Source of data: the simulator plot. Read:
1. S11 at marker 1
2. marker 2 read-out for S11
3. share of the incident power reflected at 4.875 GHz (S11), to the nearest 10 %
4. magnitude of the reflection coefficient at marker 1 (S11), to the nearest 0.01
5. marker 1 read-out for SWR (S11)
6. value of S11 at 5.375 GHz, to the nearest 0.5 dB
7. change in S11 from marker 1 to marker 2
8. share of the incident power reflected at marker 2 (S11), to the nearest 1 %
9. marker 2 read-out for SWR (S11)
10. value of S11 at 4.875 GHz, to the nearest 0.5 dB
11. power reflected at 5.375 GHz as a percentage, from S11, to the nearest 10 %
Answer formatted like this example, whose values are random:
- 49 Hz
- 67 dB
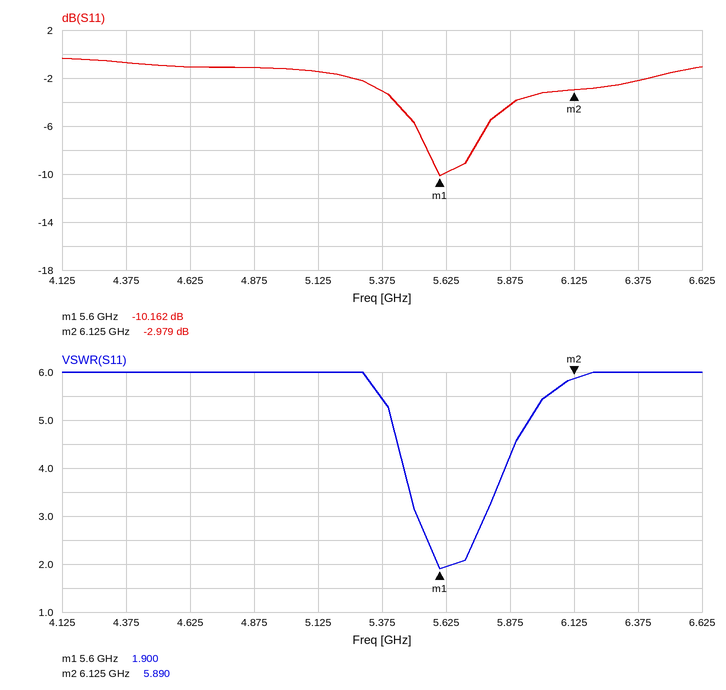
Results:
- -10.162 dB
- -2.979 dB
- 80 %
- 0.31
- 1.900
- -3.0 dB
- 7.183 dB
- 50 %
- 5.890
- -1.0 dB
- 50 %
